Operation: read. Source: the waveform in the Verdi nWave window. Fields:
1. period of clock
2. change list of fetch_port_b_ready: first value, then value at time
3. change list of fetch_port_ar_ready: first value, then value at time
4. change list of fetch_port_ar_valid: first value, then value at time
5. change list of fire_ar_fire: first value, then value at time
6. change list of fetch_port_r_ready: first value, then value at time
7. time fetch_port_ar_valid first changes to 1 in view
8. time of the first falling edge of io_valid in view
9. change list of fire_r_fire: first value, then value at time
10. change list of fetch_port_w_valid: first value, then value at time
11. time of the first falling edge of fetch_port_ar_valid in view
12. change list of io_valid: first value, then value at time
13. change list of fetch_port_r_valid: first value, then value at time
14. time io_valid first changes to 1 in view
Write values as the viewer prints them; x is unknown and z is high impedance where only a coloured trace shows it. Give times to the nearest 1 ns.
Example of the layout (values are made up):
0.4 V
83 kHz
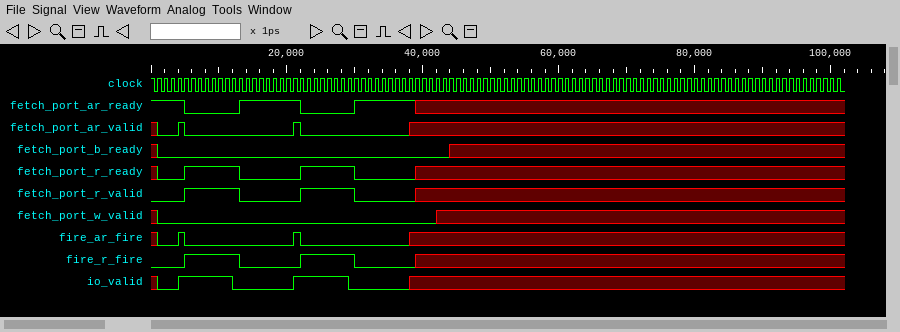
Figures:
1 ns
x, 0 at 1 ns, x at 44 ns
1, 0 at 5 ns, 1 at 13 ns, 0 at 22 ns, 1 at 30 ns, x at 39 ns
x, 0 at 1 ns, 1 at 4 ns, 0 at 5 ns, 1 at 21 ns, 0 at 22 ns, x at 38 ns
x, 0 at 1 ns, 1 at 4 ns, 0 at 5 ns, 1 at 21 ns, 0 at 22 ns, x at 38 ns
x, 0 at 1 ns, 1 at 5 ns, 0 at 13 ns, 1 at 22 ns, 0 at 30 ns, x at 39 ns
4 ns
12 ns
0, 1 at 5 ns, 0 at 13 ns, 1 at 22 ns, 0 at 30 ns, x at 39 ns
x, 0 at 1 ns, x at 42 ns
5 ns
x, 0 at 1 ns, 1 at 4 ns, 0 at 12 ns, 1 at 21 ns, 0 at 29 ns, x at 38 ns
0, 1 at 5 ns, 0 at 13 ns, 1 at 22 ns, 0 at 30 ns, x at 39 ns
4 ns
